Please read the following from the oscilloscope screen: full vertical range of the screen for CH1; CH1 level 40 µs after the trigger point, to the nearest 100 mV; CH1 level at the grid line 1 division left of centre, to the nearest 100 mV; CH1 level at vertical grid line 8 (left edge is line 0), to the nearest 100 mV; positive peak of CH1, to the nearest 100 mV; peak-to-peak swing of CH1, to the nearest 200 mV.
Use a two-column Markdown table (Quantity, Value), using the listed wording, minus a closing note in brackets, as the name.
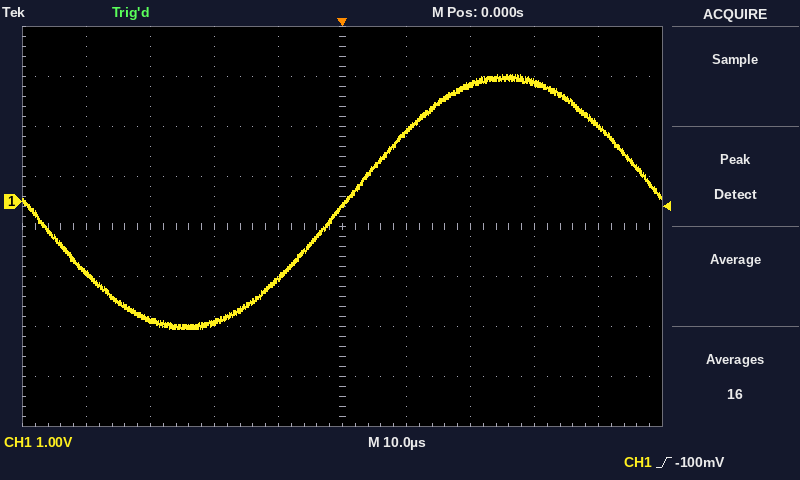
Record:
| Quantity | Value |
|---|---|
| full vertical range of the screen for CH1 | 8 V |
| CH1 level 40 µs after the trigger point, to the nearest 100 mV | 1.5 V |
| CH1 level at the grid line 1 division left of centre, to the nearest 100 mV | -1.5 V |
| CH1 level at vertical grid line 8 (left edge is line 0), to the nearest 100 mV | 2.4 V |
| positive peak of CH1, to the nearest 100 mV | 2.5 V |
| peak-to-peak swing of CH1, to the nearest 200 mV | 5.0 V |
